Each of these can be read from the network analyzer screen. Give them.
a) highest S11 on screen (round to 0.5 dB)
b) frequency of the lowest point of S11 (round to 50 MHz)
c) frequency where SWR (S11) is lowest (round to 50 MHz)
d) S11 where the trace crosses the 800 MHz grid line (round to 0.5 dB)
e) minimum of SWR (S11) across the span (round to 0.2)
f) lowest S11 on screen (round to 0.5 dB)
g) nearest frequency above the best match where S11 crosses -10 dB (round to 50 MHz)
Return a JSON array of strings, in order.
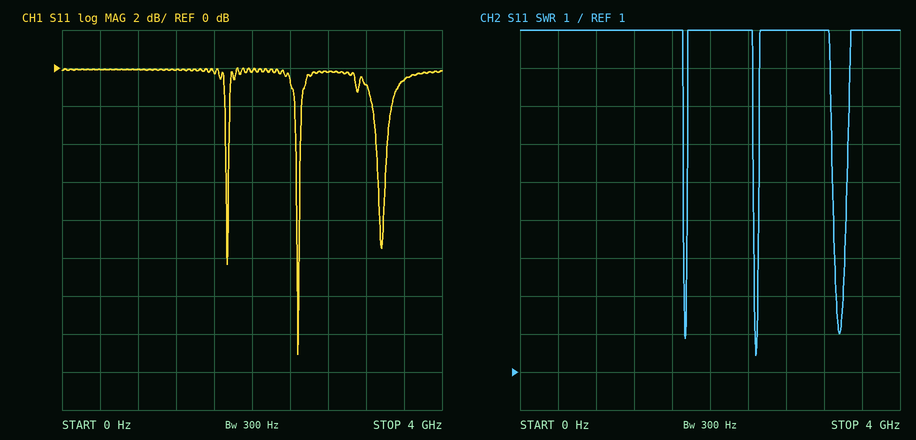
["0.0 dB", "2.50 GHz", "2.50 GHz", "0.0 dB", "1.4", "-15.0 dB", "2.50 GHz"]
